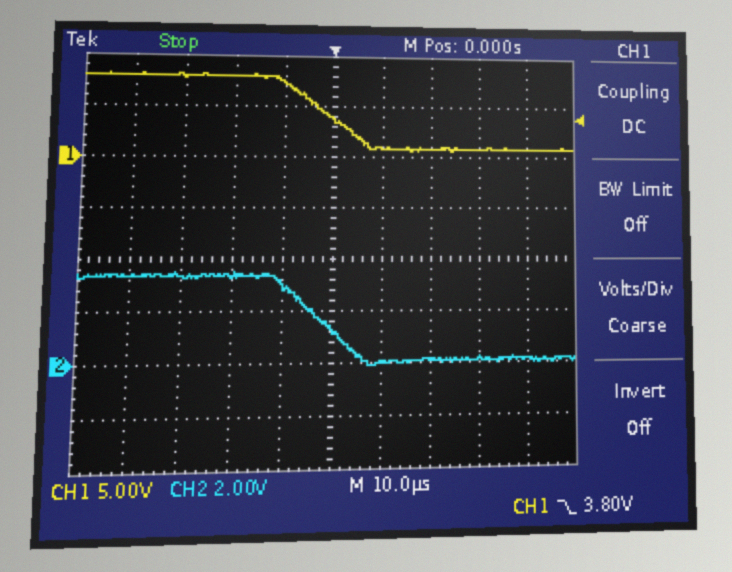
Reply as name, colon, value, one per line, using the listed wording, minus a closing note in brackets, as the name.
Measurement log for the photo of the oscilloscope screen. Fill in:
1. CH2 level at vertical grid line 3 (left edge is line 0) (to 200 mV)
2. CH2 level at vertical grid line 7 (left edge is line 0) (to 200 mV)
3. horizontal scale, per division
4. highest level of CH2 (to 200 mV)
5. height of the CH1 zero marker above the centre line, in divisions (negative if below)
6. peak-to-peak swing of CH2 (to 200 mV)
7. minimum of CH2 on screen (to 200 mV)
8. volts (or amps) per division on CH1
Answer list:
CH2 level at vertical grid line 3 (left edge is line 0): 3.4 V
CH2 level at vertical grid line 7 (left edge is line 0): 200 mV
horizontal scale, per division: 10 µs
highest level of CH2: 3.6 V
height of the CH1 zero marker above the centre line, in divisions: +2.0 div
peak-to-peak swing of CH2: 3.6 V
minimum of CH2 on screen: 0.0 V
volts (or amps) per division on CH1: 5 V
